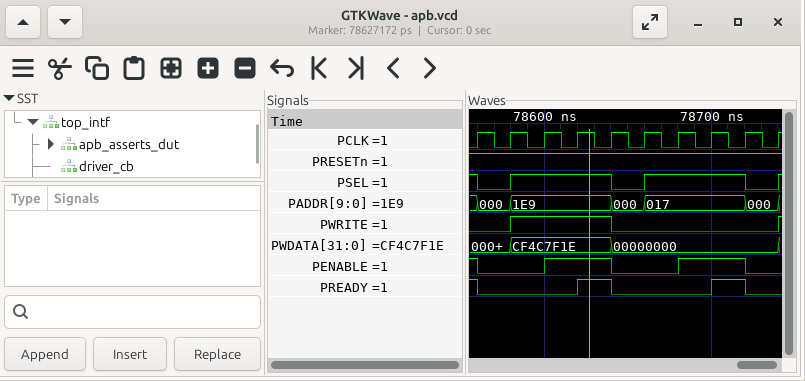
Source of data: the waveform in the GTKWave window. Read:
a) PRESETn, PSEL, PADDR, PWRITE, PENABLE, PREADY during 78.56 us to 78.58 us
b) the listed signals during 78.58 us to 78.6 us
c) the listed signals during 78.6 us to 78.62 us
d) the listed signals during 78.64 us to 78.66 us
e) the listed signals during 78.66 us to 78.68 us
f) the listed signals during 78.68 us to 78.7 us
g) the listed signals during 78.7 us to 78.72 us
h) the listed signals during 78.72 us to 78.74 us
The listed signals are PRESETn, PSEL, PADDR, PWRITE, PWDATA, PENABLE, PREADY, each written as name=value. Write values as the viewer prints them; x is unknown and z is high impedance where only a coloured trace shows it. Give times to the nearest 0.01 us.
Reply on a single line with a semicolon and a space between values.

PRESETn=1, PSEL=0, PADDR=000, PWRITE=0, PENABLE=0, PREADY=0; PRESETn=1, PSEL=1, PADDR=1E9, PWRITE=1, PWDATA=CF4C7F1E, PENABLE=0, PREADY=0; PRESETn=1, PSEL=1, PADDR=1E9, PWRITE=1, PWDATA=CF4C7F1E, PENABLE=1, PREADY=0; PRESETn=1, PSEL=0, PADDR=000, PWRITE=0, PWDATA=00000000, PENABLE=0, PREADY=0; PRESETn=1, PSEL=1, PADDR=017, PWRITE=0, PWDATA=00000000, PENABLE=0, PREADY=0; PRESETn=1, PSEL=1, PADDR=017, PWRITE=0, PWDATA=00000000, PENABLE=1, PREADY=0; PRESETn=1, PSEL=1, PADDR=017, PWRITE=0, PWDATA=00000000, PENABLE=1, PREADY=1; PRESETn=1, PSEL=0, PADDR=000, PWRITE=0, PWDATA=00000000, PENABLE=0, PREADY=0
